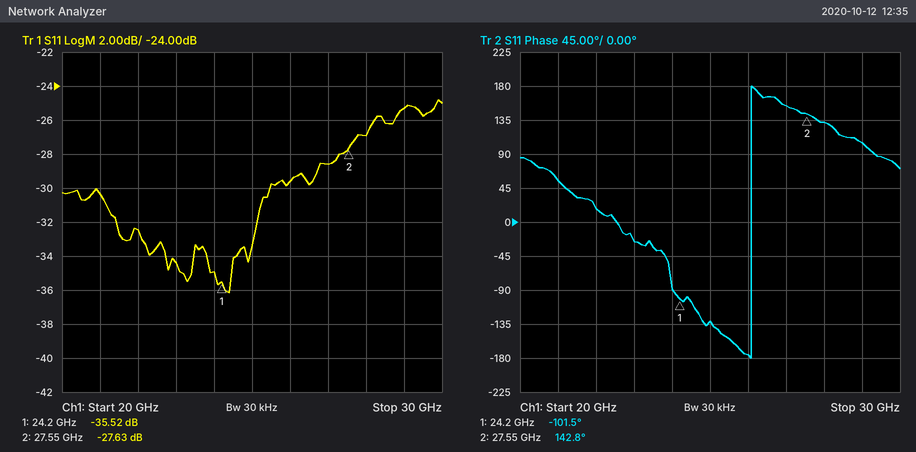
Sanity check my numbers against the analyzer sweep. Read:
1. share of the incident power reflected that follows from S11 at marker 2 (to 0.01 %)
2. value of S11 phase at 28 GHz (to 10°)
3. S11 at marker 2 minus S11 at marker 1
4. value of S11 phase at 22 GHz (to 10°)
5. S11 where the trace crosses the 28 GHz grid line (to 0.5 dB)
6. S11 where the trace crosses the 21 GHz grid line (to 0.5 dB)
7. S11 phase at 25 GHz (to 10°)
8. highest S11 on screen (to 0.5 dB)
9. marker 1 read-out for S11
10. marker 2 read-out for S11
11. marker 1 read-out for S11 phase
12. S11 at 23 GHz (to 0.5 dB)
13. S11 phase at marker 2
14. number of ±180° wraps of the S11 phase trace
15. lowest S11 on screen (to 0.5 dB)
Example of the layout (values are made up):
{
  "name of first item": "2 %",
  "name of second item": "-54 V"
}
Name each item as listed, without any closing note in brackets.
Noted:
{
  "share of the incident power reflected that follows from S11 at marker 2": "0.17 %",
  "value of S11 phase at 28 GHz": "130°",
  "S11 at marker 2 minus S11 at marker 1": "7.89 dB",
  "value of S11 phase at 22 GHz": "20°",
  "S11 where the trace crosses the 28 GHz grid line": "-27.0 dB",
  "S11 where the trace crosses the 21 GHz grid line": "-30.5 dB",
  "S11 phase at 25 GHz": "-130°",
  "highest S11 on screen": "-25.0 dB",
  "marker 1 read-out for S11": "-35.52 dB",
  "marker 2 read-out for S11": "-27.63 dB",
  "marker 1 read-out for S11 phase": "-101.5°",
  "S11 at 23 GHz": "-34.5 dB",
  "S11 phase at marker 2": "142.8°",
  "number of ±180° wraps of the S11 phase trace": "1",
  "lowest S11 on screen": "-36.0 dB"
}
